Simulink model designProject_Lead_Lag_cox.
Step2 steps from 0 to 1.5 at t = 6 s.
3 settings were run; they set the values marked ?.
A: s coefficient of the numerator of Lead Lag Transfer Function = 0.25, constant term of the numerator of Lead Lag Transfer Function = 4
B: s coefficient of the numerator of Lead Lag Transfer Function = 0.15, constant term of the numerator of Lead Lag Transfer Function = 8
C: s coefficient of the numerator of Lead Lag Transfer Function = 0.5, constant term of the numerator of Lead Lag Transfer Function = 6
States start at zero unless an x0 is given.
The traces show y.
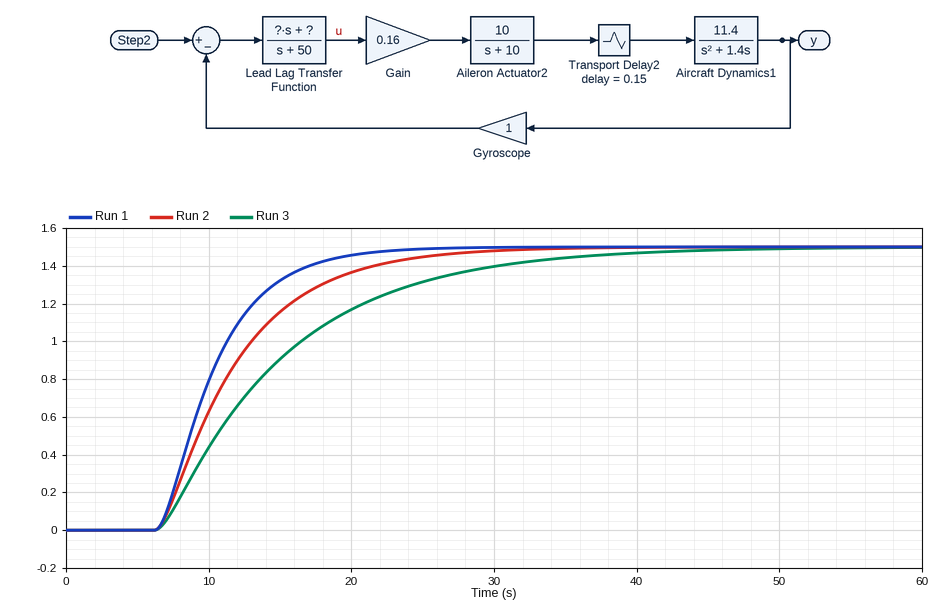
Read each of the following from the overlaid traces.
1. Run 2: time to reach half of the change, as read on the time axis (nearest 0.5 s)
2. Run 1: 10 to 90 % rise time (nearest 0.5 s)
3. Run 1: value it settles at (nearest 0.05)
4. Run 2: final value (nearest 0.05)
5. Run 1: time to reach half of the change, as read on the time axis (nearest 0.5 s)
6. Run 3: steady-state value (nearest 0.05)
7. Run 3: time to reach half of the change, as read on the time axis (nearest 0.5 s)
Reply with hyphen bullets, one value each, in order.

- 11.0 s
- 8.5 s
- 1.50
- 1.50
- 10.0 s
- 1.50
- 13.0 s
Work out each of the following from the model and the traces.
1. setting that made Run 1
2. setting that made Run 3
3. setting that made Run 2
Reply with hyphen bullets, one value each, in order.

- B
- A
- C
